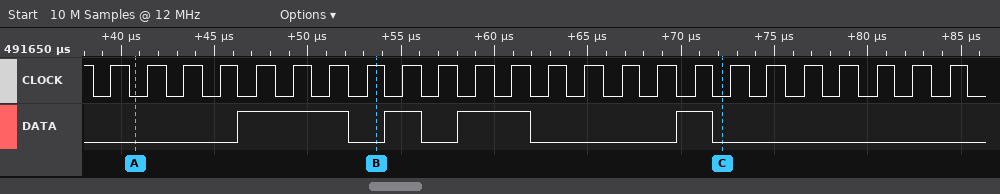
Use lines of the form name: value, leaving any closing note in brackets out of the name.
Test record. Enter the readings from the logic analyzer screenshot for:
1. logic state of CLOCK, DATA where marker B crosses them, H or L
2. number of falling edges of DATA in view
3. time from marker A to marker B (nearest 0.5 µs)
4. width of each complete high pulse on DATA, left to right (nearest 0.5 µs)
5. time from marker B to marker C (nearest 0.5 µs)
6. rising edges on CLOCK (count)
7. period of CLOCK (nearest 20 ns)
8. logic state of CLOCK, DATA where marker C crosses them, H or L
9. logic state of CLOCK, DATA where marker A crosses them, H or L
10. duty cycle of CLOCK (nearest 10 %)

logic state of CLOCK, DATA where marker B crosses them, H or L: CLOCK=H, DATA=L
number of falling edges of DATA in view: 4
time from marker A to marker B: 13 µs
width of each complete high pulse on DATA, left to right: 6 µs, 2 µs, 4 µs, 2 µs
time from marker B to marker C: 18.5 µs
rising edges on CLOCK: 24
period of CLOCK: 1960 ns
logic state of CLOCK, DATA where marker C crosses them, H or L: CLOCK=L, DATA=L
logic state of CLOCK, DATA where marker A crosses them, H or L: CLOCK=L, DATA=L
duty cycle of CLOCK: 50 %
